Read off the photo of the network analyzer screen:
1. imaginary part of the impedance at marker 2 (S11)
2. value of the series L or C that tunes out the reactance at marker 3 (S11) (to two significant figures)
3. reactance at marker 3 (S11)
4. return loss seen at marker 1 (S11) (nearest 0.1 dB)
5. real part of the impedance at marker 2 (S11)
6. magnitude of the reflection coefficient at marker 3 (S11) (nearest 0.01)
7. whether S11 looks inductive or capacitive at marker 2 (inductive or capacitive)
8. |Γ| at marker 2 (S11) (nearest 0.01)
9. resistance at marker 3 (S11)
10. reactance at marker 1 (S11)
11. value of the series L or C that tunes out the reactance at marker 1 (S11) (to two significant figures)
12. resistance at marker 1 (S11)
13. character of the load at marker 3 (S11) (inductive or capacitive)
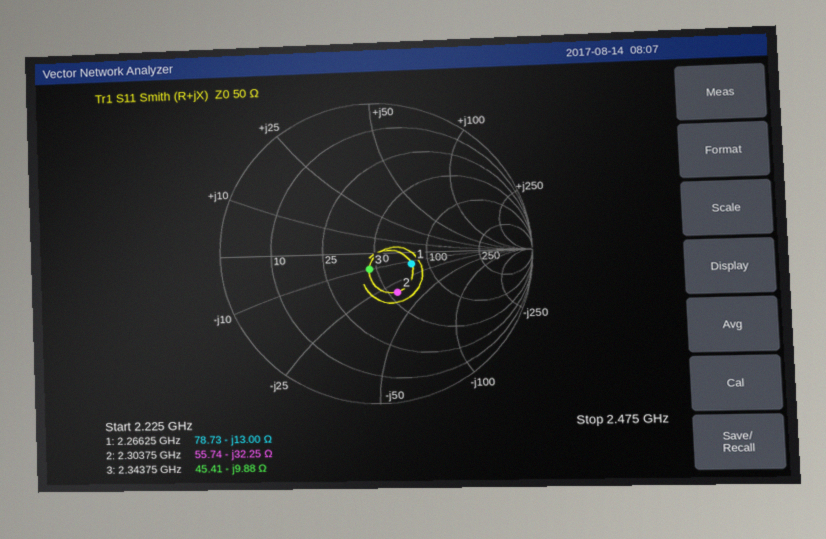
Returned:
-32.25 Ω
670 pH
-9.88 Ω
12.3 dB
55.74 Ω
0.11
capacitive
0.30
45.41 Ω
-13.00 Ω
910 pH
78.73 Ω
capacitive
